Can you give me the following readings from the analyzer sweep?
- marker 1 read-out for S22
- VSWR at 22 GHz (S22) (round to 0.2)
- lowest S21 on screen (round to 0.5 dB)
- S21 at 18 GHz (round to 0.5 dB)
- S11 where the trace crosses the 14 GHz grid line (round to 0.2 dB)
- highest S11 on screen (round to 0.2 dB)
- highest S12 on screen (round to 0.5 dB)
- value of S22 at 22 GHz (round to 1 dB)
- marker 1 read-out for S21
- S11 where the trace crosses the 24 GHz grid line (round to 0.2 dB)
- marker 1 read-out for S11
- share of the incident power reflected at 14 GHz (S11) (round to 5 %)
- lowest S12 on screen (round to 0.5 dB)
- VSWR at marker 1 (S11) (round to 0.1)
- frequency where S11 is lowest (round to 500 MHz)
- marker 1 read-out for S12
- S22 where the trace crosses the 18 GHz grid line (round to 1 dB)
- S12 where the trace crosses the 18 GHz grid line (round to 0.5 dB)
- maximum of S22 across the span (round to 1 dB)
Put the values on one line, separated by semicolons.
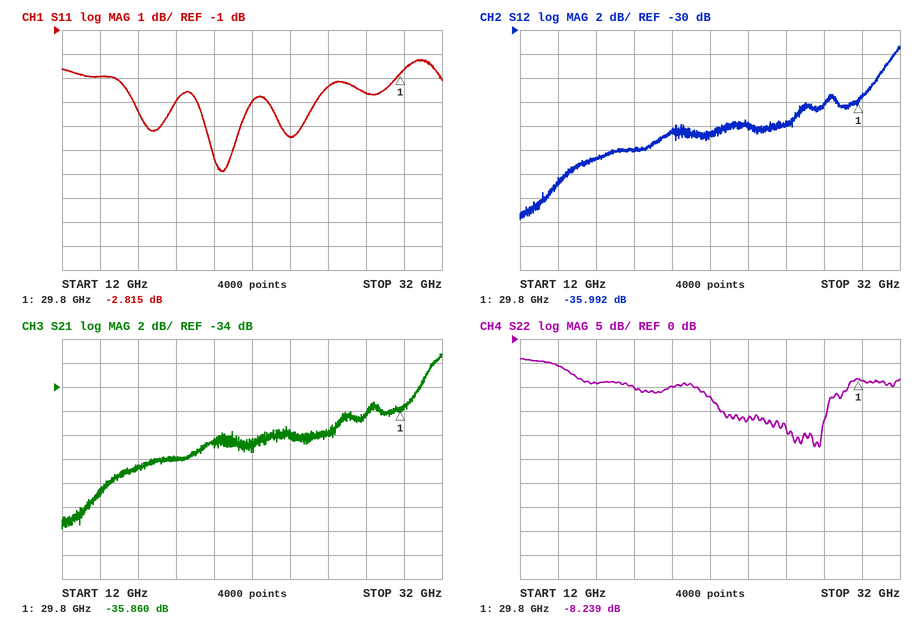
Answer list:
-8.239 dB; 1.6; -46.0 dB; -40.0 dB; -3.0 dB; -2.2 dB; -31.5 dB; -12 dB; -35.860 dB; -5.4 dB; -2.815 dB; 50 %; -46.0 dB; 6.2; 20.5 GHz; -35.992 dB; -10 dB; -40.0 dB; -4 dB
